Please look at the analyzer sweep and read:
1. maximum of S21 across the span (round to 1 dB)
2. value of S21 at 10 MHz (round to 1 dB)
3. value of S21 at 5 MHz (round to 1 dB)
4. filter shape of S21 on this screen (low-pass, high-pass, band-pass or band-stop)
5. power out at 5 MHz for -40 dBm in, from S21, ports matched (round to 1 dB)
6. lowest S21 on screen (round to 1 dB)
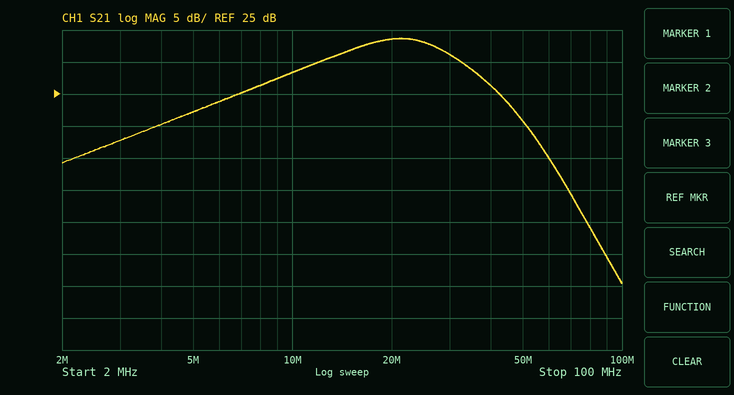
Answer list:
34 dB
28 dB
22 dB
band-pass
-18 dBm
-5 dB
